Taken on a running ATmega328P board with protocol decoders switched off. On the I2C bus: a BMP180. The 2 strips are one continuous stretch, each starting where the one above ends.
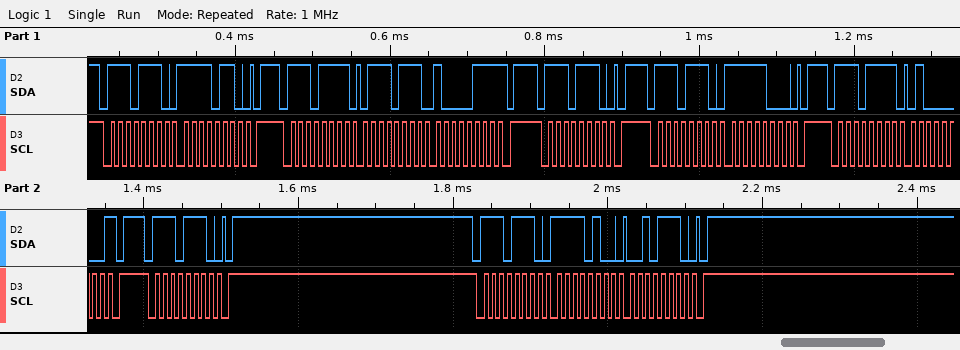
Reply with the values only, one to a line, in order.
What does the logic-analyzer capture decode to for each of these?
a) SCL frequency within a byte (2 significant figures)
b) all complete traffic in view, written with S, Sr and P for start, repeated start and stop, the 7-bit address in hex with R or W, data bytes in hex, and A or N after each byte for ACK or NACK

100 kHz
S 77W A F6 A P S 77R A 77 A 87 N P S 77W A P S 77W A F8 A P S 77R A 40 N P S 77W A P S 77W A F4 A 2E A P
